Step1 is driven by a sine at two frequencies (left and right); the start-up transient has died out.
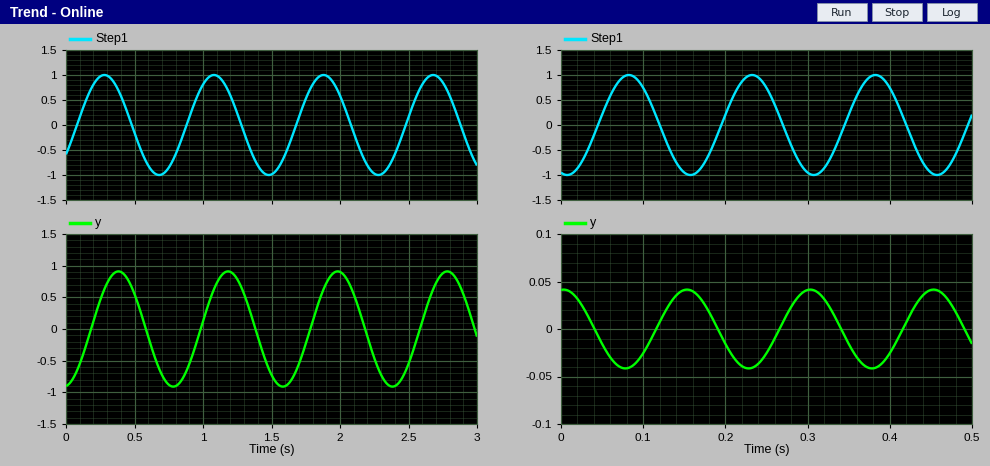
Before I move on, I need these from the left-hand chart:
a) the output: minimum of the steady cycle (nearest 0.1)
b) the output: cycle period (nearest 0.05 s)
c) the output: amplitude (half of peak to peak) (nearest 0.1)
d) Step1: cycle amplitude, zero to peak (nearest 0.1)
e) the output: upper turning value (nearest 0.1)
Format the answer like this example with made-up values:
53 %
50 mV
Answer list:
-0.9
0.80 s
0.9
1.0
0.9
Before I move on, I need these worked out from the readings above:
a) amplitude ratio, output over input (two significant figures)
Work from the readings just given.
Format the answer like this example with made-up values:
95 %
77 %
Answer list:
0.90
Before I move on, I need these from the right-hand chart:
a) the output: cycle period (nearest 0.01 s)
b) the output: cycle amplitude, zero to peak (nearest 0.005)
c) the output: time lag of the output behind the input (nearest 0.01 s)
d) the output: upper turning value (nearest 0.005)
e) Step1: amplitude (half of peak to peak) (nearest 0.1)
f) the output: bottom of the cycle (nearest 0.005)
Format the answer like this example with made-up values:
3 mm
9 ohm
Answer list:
0.15 s
0.040
0.07 s
0.040
1.0
-0.040
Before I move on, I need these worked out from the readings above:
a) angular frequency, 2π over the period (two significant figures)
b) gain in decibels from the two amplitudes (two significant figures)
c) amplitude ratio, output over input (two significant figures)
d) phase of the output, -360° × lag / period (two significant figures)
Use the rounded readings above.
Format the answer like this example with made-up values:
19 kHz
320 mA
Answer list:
42 rad/s
-28 dB
0.040
-170°
